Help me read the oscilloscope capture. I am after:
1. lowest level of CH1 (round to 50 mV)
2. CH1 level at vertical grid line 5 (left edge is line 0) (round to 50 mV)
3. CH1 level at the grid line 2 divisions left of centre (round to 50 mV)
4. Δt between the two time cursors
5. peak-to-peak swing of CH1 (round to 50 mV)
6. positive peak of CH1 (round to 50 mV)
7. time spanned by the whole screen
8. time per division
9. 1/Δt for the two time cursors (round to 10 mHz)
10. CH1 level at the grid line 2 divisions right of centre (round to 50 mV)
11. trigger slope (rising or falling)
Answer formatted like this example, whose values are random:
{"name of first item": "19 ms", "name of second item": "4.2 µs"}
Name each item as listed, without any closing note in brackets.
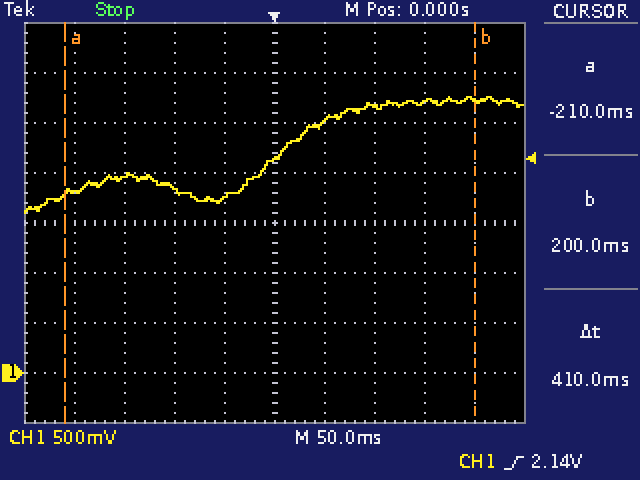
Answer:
{"lowest level of CH1": "1.60 V", "CH1 level at vertical grid line 5 (left edge is line 0)": "2.15 V", "CH1 level at the grid line 2 divisions left of centre": "1.85 V", "Δt between the two time cursors": "410 ms", "peak-to-peak swing of CH1": "1.15 V", "positive peak of CH1": "2.75 V", "time spanned by the whole screen": "500 ms", "time per division": "50 ms", "1/Δt for the two time cursors": "2.44 Hz", "CH1 level at the grid line 2 divisions right of centre": "2.65 V", "trigger slope": "rising"}
